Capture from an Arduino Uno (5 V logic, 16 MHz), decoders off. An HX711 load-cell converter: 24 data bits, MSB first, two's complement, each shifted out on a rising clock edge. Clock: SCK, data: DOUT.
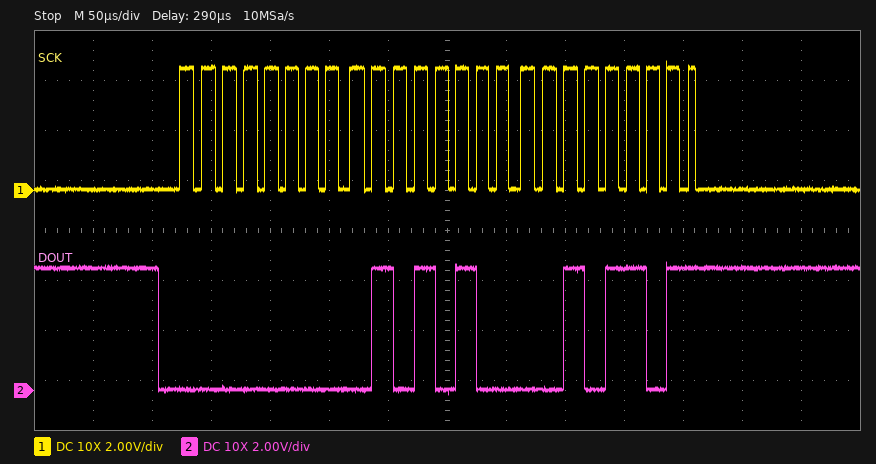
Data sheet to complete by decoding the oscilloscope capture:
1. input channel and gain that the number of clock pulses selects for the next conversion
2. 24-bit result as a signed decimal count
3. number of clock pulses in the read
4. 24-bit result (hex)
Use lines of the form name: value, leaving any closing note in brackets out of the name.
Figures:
input channel and gain that the number of clock pulses selects for the next conversion: channel A, gain 128
24-bit result as a signed decimal count: 21549
number of clock pulses in the read: 25
24-bit result: 0x00542D
